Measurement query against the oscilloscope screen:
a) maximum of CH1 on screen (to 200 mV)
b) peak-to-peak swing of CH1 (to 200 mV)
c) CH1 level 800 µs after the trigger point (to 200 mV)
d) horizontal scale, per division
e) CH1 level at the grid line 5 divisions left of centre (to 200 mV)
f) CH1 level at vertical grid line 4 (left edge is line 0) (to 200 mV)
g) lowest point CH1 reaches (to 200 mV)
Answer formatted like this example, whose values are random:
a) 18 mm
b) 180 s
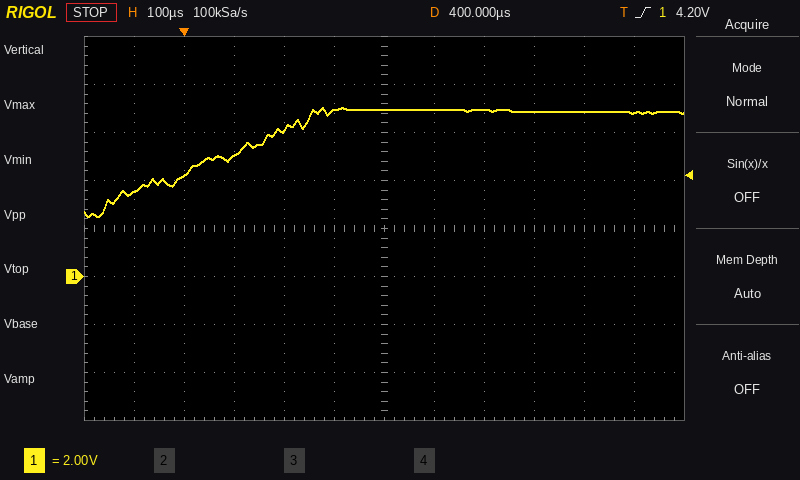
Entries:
a) 7.0 V
b) 4.6 V
c) 6.8 V
d) 100 µs
e) 3.6 V
f) 6.2 V
g) 2.4 V
